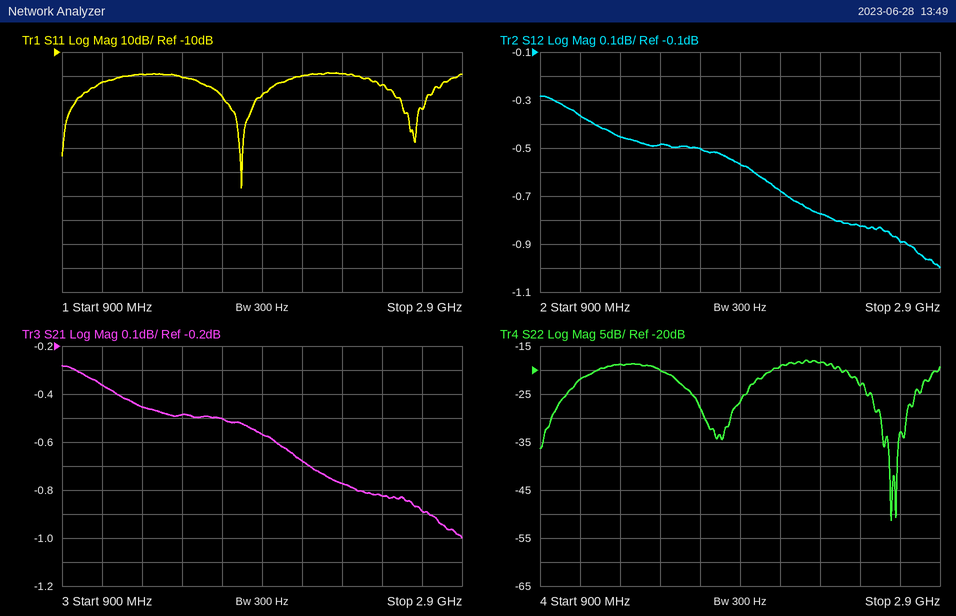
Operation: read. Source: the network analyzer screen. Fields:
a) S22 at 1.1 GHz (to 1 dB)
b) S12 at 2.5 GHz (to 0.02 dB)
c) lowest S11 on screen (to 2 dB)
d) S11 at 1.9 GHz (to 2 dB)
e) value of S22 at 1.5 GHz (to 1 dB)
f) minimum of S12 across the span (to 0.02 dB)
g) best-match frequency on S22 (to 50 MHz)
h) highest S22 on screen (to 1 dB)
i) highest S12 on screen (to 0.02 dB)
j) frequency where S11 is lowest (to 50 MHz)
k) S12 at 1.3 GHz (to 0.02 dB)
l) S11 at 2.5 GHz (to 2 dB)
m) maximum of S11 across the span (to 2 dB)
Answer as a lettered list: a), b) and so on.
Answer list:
a) -22 dB
b) -0.82 dB
c) -66 dB
d) -28 dB
e) -20 dB
f) -1.00 dB
g) 2.65 GHz
h) -18 dB
i) -0.28 dB
j) 1.80 GHz
k) -0.46 dB
l) -24 dB
m) -18 dB
